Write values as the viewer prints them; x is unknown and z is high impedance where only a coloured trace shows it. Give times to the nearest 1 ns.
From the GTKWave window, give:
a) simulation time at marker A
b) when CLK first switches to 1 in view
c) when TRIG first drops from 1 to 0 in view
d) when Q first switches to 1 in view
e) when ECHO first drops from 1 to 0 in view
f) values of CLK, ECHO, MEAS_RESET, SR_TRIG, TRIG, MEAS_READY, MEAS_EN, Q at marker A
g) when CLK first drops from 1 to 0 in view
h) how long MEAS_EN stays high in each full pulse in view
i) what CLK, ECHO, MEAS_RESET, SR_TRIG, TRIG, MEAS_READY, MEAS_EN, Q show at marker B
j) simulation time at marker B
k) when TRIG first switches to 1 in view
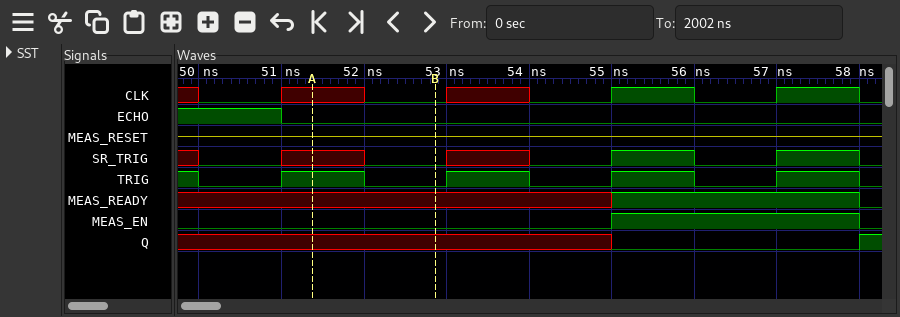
51 ns
55 ns
50 ns
58 ns
51 ns
CLK=x, ECHO=0, MEAS_RESET=z, SR_TRIG=x, TRIG=1, MEAS_READY=x, MEAS_EN=0, Q=x
56 ns
3 ns
CLK=0, ECHO=0, MEAS_RESET=z, SR_TRIG=0, TRIG=0, MEAS_READY=x, MEAS_EN=0, Q=x
53 ns
51 ns
